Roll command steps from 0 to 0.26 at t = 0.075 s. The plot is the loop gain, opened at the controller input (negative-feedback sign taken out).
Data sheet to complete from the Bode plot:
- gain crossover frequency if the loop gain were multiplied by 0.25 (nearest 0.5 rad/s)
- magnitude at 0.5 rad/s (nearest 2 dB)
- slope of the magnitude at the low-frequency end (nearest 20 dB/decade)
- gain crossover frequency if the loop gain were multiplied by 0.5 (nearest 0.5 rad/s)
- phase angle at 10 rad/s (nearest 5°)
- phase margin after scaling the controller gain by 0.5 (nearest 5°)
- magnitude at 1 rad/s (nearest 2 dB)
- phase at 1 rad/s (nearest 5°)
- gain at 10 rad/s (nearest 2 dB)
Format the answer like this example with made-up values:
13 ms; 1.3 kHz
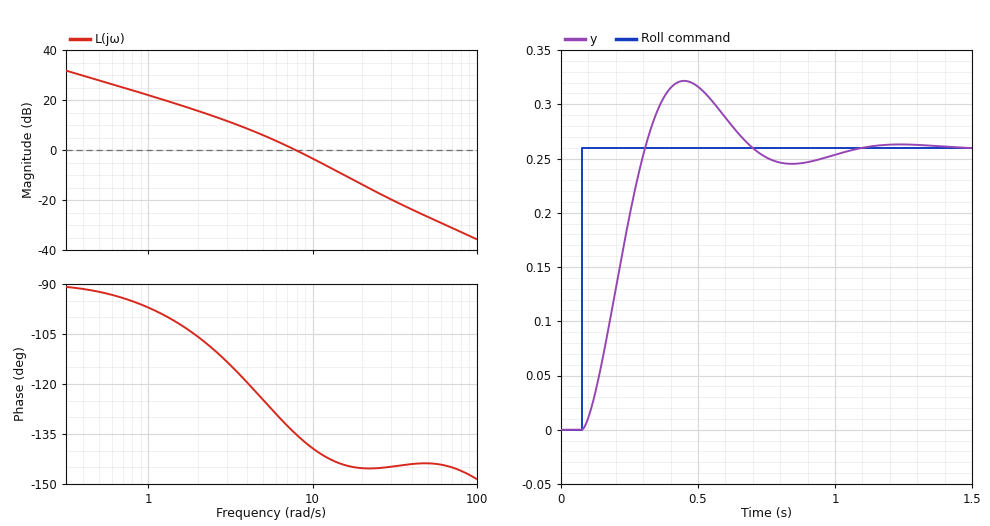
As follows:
3.0 rad/s; 28 dB; -20 dB/decade; 5.0 rad/s; -140°; 55°; 22 dB; -95°; -4 dB
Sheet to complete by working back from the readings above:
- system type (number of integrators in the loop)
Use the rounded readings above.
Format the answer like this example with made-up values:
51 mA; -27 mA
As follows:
1
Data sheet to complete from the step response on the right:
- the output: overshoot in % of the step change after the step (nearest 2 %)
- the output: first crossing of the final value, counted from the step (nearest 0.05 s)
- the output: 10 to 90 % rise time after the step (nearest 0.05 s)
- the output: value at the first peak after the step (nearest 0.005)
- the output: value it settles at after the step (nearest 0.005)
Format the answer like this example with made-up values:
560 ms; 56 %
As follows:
24 %; 0.25 s; 0.15 s; 0.320; 0.260
